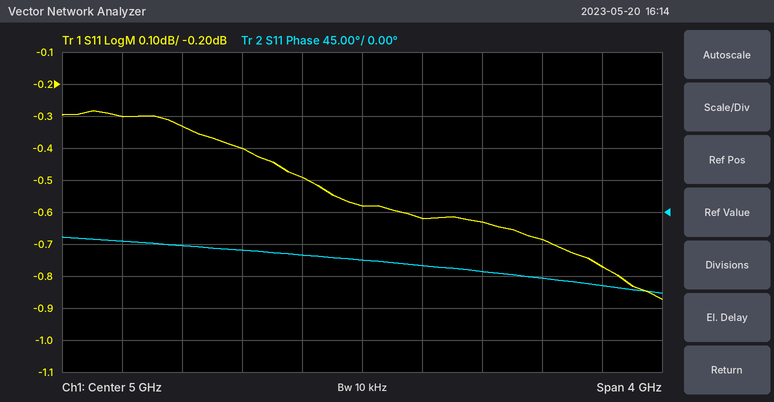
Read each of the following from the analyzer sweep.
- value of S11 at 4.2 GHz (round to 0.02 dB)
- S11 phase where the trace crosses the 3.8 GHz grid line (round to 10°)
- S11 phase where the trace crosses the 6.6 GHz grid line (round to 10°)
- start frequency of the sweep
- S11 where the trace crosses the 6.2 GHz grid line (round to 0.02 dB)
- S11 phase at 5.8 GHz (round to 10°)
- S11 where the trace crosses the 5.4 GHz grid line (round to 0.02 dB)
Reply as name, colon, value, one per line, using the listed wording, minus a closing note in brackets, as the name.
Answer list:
value of S11 at 4.2 GHz: -0.40 dB
S11 phase where the trace crosses the 3.8 GHz grid line: -50°
S11 phase where the trace crosses the 6.6 GHz grid line: -100°
start frequency of the sweep: 3 GHz
S11 where the trace crosses the 6.2 GHz grid line: -0.68 dB
S11 phase at 5.8 GHz: -80°
S11 where the trace crosses the 5.4 GHz grid line: -0.62 dB
